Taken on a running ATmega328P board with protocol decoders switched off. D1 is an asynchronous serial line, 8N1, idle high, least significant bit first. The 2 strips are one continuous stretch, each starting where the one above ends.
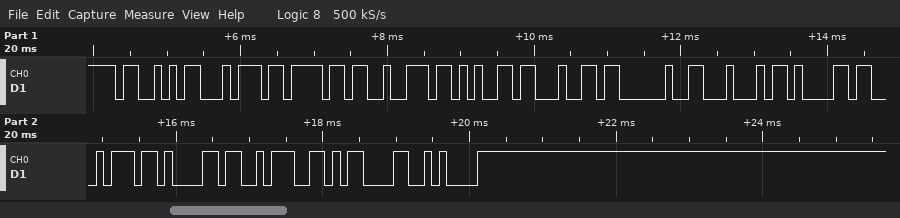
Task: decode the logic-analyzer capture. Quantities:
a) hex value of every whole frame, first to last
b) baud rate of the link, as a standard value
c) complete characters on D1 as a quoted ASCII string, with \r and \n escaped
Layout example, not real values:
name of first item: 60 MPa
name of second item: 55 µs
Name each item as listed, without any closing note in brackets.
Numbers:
hex value of every whole frame, first to last: 0x53 0x74 0x6F 0x72 0x65 0x64 0x20 0x44 0x61 0x74 0x61 0x3A 0x0D 0x0A
baud rate of the link, as a standard value: 9600 baud
complete characters on D1 as a quoted ASCII string, with \r and \n escaped: "Stored Data:\r\n"
